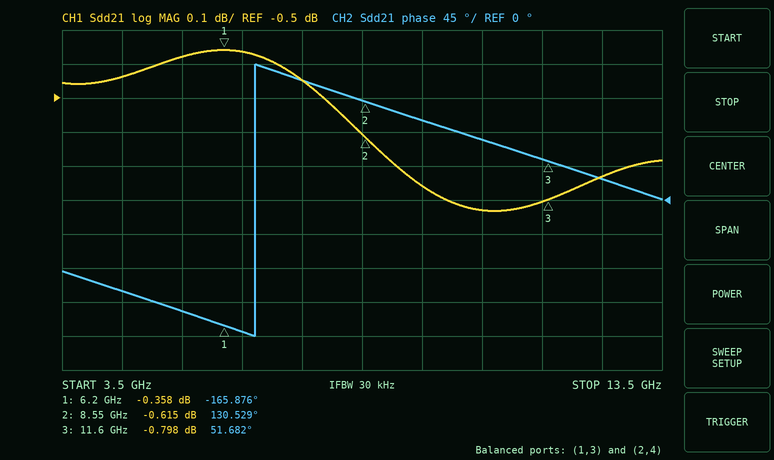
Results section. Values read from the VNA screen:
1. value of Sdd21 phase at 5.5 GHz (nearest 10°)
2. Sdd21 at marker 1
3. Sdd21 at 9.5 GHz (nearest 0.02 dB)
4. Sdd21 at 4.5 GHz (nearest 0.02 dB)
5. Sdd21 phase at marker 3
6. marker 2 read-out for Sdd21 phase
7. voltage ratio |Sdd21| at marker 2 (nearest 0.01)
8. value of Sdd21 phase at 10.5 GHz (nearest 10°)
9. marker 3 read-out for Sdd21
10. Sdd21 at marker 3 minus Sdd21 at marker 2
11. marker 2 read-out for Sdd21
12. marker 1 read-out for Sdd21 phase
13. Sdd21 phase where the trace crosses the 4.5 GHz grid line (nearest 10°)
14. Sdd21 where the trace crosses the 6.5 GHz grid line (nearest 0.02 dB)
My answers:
-150°
-0.358 dB
-0.76 dB
-0.44 dB
51.682°
130.529°
0.93
80°
-0.798 dB
-0.183 dB
-0.615 dB
-165.876°
-120°
-0.36 dB
